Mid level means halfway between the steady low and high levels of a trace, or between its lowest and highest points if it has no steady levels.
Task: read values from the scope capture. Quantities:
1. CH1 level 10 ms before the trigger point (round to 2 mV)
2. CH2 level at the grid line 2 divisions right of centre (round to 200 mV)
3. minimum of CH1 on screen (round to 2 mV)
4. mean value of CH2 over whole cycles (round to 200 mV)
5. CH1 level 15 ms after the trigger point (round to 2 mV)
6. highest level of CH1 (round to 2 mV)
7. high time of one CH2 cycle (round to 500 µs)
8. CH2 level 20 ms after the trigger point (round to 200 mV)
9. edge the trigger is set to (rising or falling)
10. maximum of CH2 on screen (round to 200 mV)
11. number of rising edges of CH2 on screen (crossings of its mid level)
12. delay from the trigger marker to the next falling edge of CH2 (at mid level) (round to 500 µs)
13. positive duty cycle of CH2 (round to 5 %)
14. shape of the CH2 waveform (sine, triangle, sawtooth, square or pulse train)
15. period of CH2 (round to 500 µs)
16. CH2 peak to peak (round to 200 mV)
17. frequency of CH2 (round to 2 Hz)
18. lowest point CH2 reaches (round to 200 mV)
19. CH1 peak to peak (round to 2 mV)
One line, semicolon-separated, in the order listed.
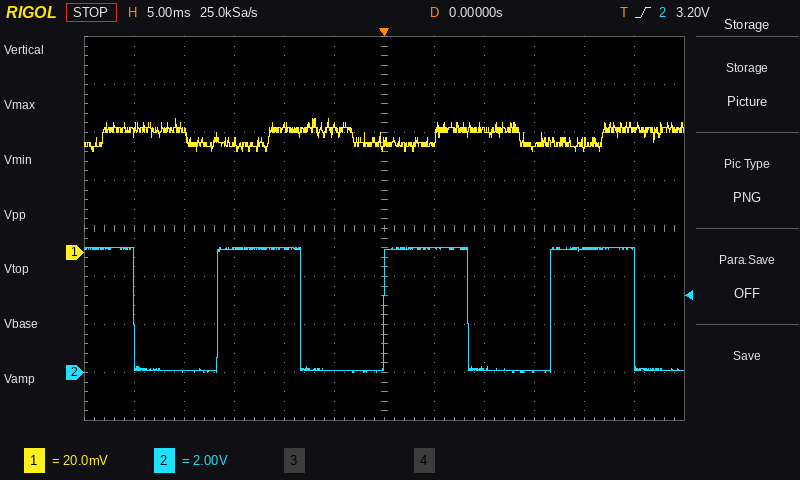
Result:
52 mV; 200 mV; 42 mV; 2.6 V; 44 mV; 56 mV; 8.5 ms; 5.2 V; rising; 5.2 V; 3; 8.5 ms; 50 %; square; 16.5 ms; 5.2 V; 60 Hz; 0.0 V; 14 mV
